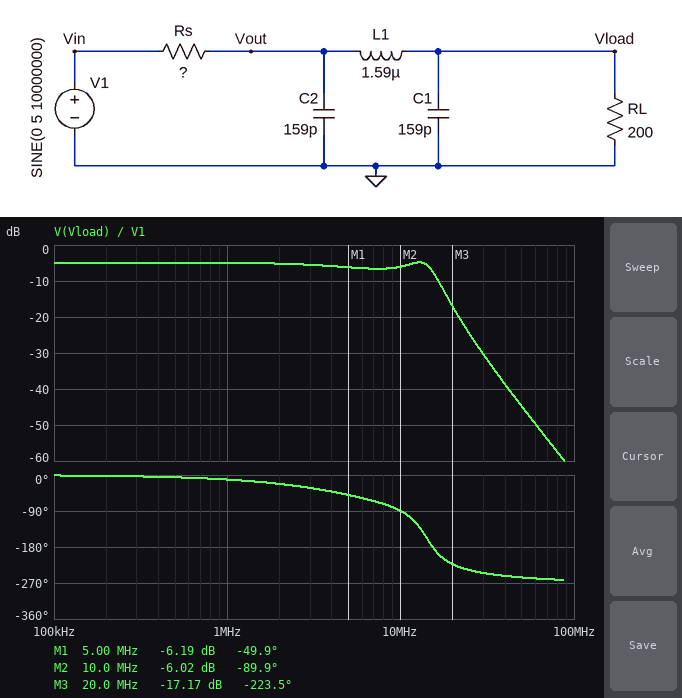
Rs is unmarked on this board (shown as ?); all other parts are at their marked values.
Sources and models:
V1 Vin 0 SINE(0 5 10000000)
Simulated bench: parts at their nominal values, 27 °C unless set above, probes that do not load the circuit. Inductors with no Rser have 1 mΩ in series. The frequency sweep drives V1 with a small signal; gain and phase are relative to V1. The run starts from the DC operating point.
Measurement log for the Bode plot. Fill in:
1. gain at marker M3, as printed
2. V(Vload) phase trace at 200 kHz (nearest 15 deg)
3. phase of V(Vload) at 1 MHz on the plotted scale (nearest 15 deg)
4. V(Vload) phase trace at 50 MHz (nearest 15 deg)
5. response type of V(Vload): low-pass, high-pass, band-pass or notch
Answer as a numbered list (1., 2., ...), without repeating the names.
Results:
1. -17.17 dB
2. 0 deg
3. -15 deg
4. -255 deg
5. low-pass
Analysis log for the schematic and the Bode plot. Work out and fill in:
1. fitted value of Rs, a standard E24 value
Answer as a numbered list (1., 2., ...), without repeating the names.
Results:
1. 150 Ω
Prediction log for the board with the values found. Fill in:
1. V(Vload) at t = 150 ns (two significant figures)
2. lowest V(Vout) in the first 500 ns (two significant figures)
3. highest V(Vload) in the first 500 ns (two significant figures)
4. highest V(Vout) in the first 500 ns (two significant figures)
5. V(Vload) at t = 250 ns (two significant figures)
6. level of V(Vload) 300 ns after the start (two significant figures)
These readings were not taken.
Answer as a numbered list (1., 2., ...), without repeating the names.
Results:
1. 2.6 V
2. -1.5 V
3. 2.6 V
4. 2.1 V
5. 2.5 V
6. -2.5 V
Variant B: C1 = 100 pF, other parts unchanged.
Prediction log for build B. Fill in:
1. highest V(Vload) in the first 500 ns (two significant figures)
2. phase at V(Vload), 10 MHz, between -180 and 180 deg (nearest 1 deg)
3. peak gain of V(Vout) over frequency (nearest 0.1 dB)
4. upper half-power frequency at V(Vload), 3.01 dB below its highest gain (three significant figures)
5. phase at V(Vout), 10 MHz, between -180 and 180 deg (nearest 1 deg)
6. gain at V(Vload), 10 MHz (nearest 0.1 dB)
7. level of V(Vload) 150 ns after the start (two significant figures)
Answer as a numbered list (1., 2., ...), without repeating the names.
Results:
1. 2.5 V
2. -79 deg
3. -4.9 dB
4. 17.5 MHz
5. -26 deg
6. -6.2 dB
7. 2.4 V
